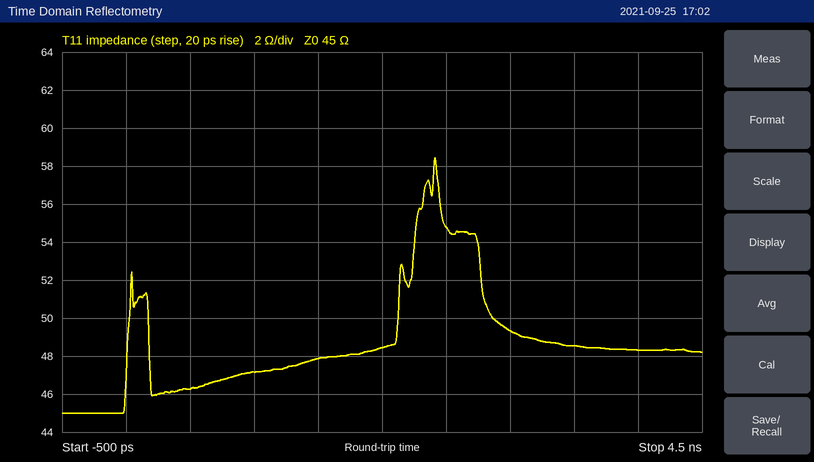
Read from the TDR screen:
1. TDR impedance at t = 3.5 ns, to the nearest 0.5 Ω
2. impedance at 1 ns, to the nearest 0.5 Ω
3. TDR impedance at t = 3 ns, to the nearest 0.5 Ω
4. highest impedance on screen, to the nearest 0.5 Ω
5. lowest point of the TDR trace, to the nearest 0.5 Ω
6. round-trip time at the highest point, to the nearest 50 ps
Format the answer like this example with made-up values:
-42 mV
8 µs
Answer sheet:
48.5 Ω
47.0 Ω
49.5 Ω
58.5 Ω
45.0 Ω
2.40 ns
